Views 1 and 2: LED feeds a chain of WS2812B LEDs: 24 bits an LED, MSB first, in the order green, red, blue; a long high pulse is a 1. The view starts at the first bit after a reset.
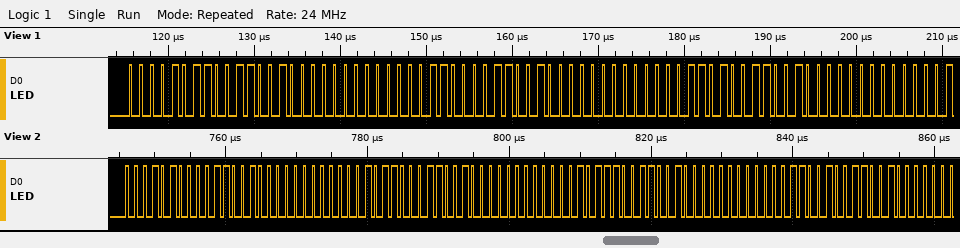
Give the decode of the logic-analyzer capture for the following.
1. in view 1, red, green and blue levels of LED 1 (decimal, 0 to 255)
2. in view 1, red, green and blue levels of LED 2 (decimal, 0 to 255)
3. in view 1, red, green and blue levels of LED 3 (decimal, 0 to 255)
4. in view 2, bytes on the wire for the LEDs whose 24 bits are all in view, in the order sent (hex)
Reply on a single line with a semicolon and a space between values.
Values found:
50, 11, 0; 50, 12, 0; 50, 13, 0; 14 32 00 16 32 00 17 32 00
